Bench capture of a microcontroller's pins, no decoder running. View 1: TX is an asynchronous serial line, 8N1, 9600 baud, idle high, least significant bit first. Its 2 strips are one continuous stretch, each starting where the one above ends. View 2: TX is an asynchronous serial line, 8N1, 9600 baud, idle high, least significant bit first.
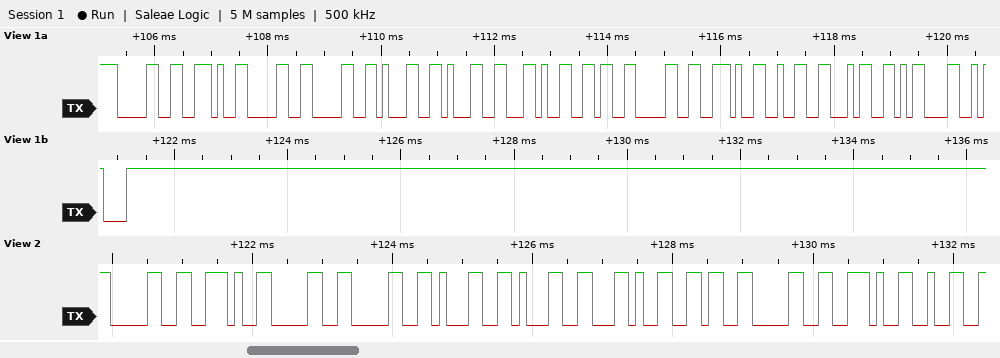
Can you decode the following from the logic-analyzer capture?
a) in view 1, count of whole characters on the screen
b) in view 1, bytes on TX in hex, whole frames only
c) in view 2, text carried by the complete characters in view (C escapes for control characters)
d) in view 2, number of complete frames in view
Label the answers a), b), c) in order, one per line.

a) 14
b) 0x30 0x2E 0x30 0x30 0x31 0x31 0x2C 0x36 0x30 0x2E 0x32 0x34 0x0D 0x0A
c) "0.0011,60.2"
d) 11
